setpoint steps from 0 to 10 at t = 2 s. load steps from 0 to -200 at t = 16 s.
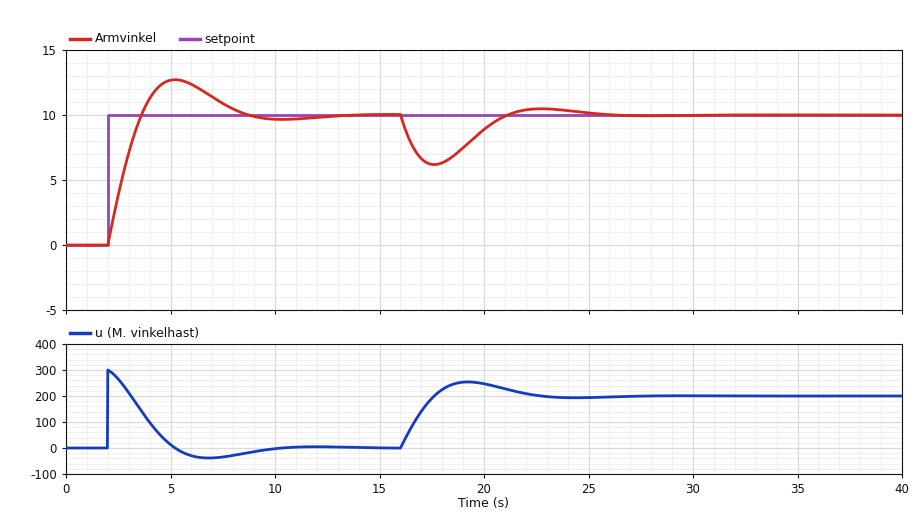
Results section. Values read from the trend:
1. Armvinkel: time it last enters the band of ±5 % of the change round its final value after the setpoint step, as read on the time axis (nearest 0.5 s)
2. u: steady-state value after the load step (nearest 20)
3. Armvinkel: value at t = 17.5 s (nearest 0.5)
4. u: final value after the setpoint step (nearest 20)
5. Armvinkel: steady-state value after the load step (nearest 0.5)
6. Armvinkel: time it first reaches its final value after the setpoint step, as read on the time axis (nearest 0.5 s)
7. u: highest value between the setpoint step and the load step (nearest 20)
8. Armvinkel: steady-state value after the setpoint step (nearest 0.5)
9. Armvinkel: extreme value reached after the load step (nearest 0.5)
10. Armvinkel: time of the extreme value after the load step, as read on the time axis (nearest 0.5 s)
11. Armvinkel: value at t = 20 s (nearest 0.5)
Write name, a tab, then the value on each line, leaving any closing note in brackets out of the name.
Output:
Armvinkel: time it last enters the band of ±5 % of the change round its final value after the setpoint step, as read on the time axis	8.0 s
u: steady-state value after the load step	200
Armvinkel: value at t = 17.5 s	6.0
u: final value after the setpoint step	0
Armvinkel: steady-state value after the load step	10.0
Armvinkel: time it first reaches its final value after the setpoint step, as read on the time axis	3.5 s
u: highest value between the setpoint step and the load step	300
Armvinkel: steady-state value after the setpoint step	10.0
Armvinkel: extreme value reached after the load step	6.0
Armvinkel: time of the extreme value after the load step, as read on the time axis	17.5 s
Armvinkel: value at t = 20 s	9.0
